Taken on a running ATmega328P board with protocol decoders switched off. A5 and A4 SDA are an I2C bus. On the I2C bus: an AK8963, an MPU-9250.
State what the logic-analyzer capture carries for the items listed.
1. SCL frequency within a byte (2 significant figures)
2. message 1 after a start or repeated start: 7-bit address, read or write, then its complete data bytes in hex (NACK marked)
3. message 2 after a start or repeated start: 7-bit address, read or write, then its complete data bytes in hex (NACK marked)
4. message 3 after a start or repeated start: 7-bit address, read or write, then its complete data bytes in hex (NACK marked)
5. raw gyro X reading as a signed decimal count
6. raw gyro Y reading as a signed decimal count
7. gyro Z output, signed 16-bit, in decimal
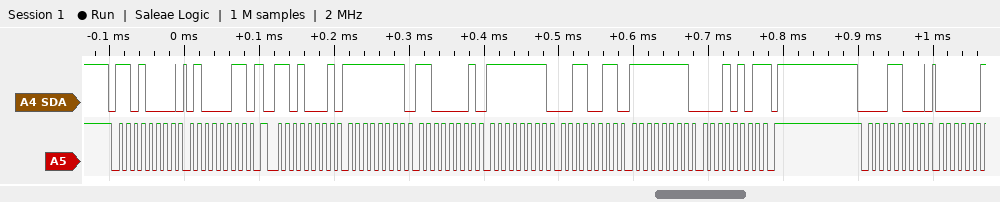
100 kHz
0x68 write: 43
0x68 read: FF C1 FF 33 FF 15 NACK
0x0C write
-63
-205
-235
